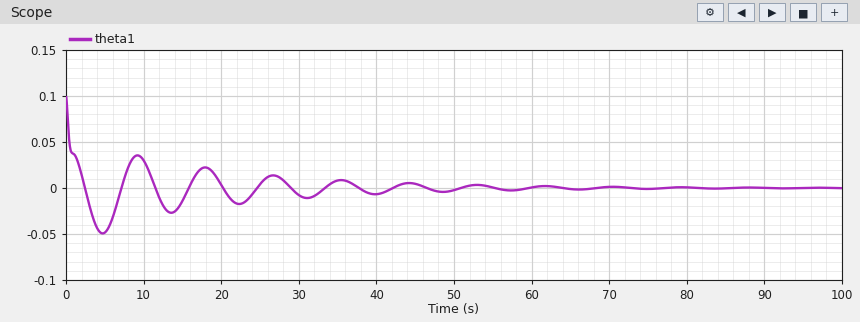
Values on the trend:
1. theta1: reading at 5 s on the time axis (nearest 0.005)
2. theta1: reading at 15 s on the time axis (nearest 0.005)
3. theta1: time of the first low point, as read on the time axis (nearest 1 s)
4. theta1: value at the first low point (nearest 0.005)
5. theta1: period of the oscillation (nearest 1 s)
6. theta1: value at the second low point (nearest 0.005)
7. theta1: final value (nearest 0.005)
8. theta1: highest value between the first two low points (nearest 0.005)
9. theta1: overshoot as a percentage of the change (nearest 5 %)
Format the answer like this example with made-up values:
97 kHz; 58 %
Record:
-0.050; -0.015; 5 s; -0.050; 9 s; -0.025; 0.000; 0.035; 50 %
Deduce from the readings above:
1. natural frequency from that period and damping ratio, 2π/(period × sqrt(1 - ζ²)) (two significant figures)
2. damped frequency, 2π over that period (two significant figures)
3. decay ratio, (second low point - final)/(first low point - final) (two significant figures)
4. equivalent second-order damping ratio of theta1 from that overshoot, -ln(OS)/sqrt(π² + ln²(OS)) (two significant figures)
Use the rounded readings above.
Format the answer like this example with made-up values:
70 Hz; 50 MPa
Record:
0.72 rad/s; 0.70 rad/s; 0.50; 0.22
